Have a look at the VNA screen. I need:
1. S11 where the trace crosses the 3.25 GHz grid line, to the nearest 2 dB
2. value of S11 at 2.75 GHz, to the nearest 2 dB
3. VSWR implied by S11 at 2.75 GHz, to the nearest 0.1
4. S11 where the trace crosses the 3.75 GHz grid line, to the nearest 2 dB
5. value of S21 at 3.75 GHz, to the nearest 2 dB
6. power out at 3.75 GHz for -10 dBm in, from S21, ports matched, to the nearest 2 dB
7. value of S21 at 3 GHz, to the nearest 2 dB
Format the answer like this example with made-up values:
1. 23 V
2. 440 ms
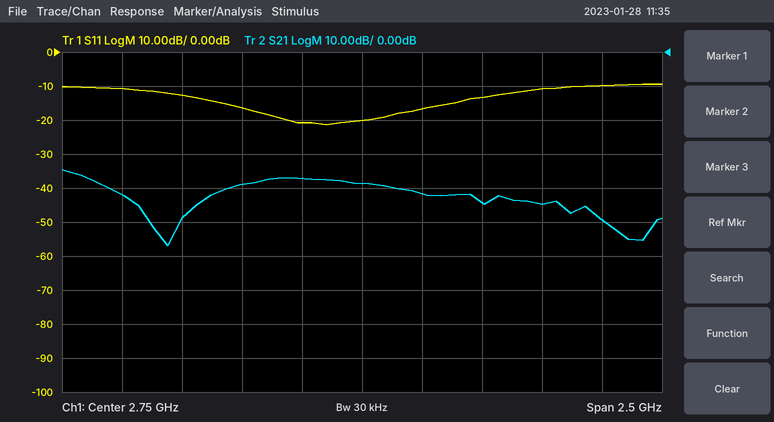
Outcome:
1. -14 dB
2. -20 dB
3. 1.2
4. -10 dB
5. -50 dB
6. -60 dBm
7. -42 dB
